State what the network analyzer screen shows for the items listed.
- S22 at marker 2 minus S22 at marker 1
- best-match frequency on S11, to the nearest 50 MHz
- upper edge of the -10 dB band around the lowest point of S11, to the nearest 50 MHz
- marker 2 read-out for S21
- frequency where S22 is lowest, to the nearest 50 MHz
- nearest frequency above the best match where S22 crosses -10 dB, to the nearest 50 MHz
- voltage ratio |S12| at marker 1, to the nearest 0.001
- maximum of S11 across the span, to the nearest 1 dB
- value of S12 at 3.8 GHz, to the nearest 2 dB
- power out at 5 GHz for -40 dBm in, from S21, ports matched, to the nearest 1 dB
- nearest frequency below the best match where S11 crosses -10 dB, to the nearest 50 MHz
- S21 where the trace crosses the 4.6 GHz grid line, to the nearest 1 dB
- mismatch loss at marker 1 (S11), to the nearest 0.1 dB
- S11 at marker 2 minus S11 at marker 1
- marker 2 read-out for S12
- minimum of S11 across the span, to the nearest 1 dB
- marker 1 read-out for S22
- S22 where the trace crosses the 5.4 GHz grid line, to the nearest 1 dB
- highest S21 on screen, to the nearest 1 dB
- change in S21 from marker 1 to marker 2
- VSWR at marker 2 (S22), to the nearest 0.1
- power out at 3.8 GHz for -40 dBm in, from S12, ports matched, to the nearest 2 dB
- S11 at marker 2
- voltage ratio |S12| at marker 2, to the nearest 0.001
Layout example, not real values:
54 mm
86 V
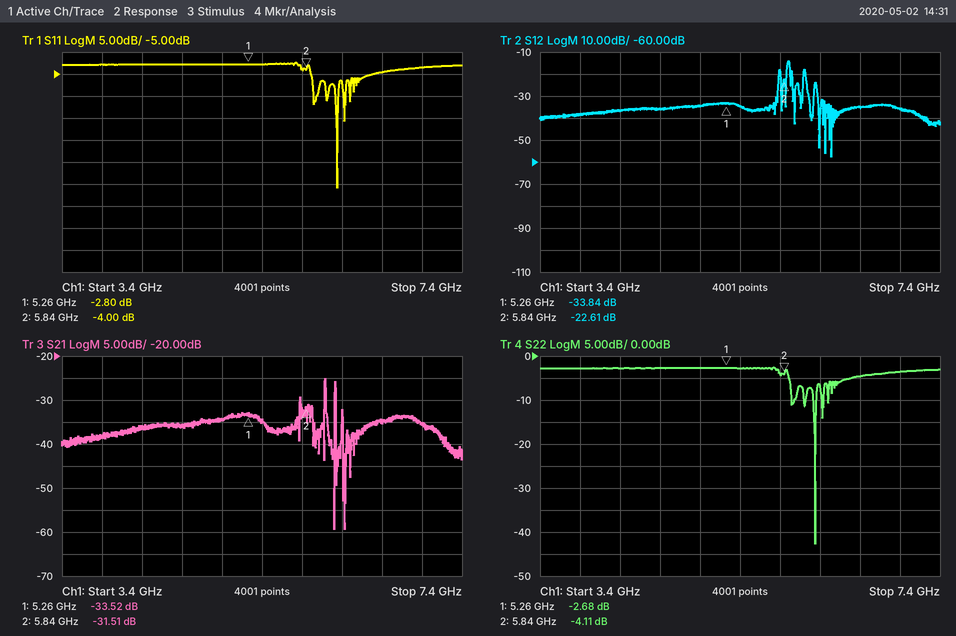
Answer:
-1.43 dB
6.15 GHz
6.15 GHz
-31.51 dB
6.15 GHz
6.15 GHz
0.020
-2 dB
-38 dB
-74 dBm
6.15 GHz
-36 dB
3.2 dB
-1.20 dB
-22.61 dB
-31 dB
-2.68 dB
-3 dB
-25 dB
2.01 dB
4.3
-78 dBm
-4.00 dB
0.074
